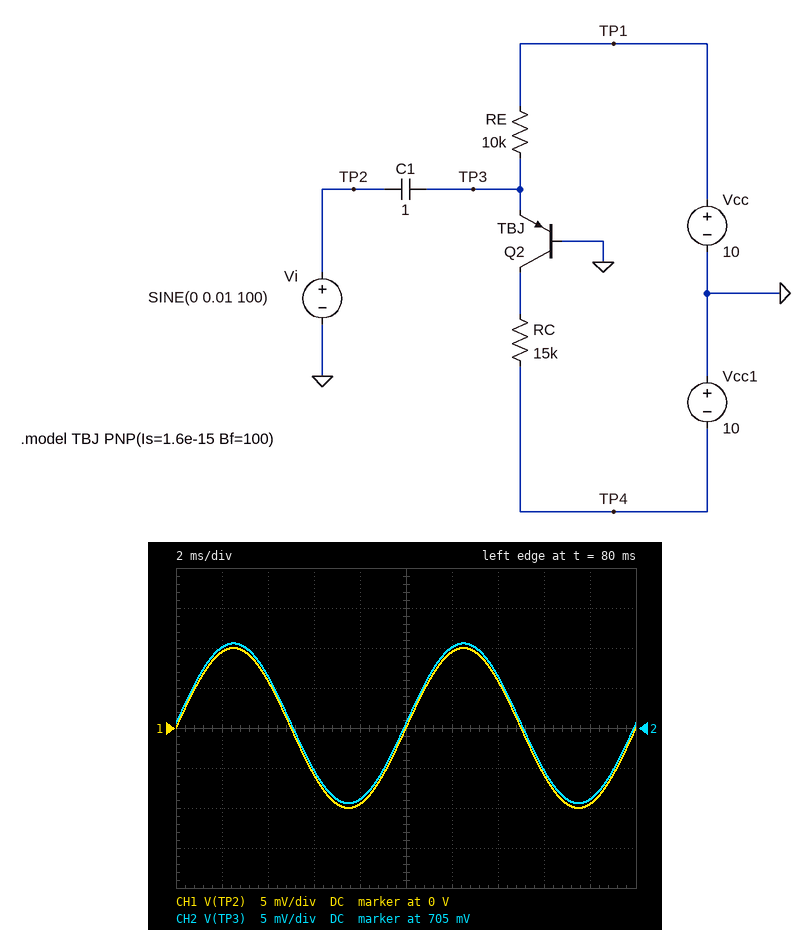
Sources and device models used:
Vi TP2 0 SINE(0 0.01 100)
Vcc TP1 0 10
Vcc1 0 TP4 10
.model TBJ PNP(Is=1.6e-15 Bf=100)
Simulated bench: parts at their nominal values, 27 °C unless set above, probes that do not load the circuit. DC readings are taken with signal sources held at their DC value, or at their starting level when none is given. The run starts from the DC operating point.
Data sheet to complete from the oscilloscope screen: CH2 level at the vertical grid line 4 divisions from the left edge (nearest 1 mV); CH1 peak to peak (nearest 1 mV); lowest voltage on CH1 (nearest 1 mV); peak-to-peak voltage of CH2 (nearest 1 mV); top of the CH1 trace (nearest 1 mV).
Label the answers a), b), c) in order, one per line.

a) 696 mV
b) 20 mV
c) -10 mV
d) 20 mV
e) 10 mV
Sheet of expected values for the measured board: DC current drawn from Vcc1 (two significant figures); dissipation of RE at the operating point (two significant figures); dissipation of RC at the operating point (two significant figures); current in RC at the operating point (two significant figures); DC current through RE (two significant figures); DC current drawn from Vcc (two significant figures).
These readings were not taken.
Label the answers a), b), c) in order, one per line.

a) 710 µA
b) 8.6 mW
c) 7.6 mW
d) 710 µA
e) 930 µA
f) 930 µA
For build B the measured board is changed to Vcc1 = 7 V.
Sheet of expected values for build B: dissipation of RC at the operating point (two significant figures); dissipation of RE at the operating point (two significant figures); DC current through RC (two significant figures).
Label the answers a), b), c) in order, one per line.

a) 3.9 mW
b) 8.6 mW
c) 510 µA
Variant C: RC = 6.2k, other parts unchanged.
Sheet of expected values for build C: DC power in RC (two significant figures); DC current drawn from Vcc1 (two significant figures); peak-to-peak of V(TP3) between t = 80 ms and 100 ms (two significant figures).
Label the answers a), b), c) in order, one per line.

a) 5.3 mW
b) 920 µA
c) 20 mV
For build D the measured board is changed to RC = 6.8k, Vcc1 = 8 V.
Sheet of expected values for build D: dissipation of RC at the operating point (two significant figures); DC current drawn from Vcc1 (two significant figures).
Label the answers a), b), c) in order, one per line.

a) 5.8 mW
b) 920 µA
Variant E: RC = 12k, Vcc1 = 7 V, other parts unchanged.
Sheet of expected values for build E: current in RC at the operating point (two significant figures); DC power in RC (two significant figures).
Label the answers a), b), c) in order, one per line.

a) 640 µA
b) 4.9 mW
